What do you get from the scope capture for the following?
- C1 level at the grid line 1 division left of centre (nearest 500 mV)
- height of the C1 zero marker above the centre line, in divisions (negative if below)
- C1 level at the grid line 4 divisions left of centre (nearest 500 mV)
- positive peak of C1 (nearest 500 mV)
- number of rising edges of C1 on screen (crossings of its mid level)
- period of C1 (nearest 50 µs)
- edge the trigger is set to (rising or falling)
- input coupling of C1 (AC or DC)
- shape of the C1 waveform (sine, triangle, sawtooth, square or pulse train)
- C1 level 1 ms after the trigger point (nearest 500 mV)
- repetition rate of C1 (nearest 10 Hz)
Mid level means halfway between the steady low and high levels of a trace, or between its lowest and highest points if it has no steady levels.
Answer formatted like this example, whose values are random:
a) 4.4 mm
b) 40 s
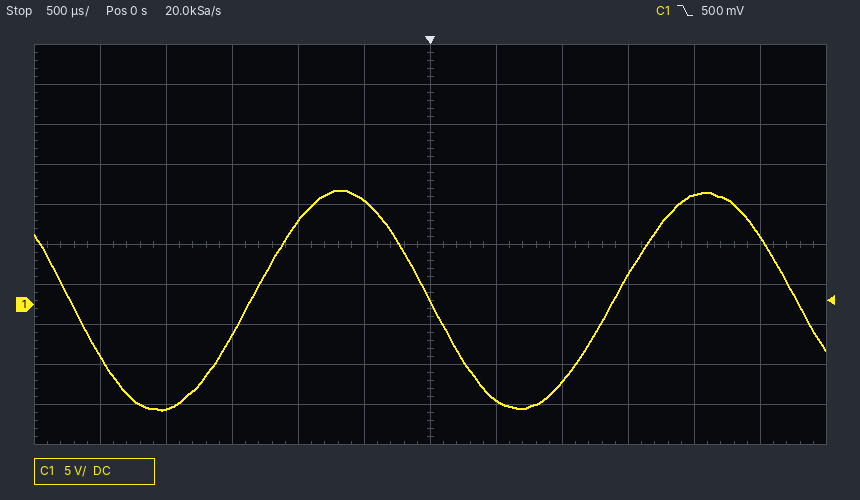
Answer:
a) 13.0 V
b) -1.5 div
c) -13.0 V
d) 14.0 V
e) 2
f) 2.75 ms
g) falling
h) DC
i) sine
j) -9.5 V
k) 360 Hz
